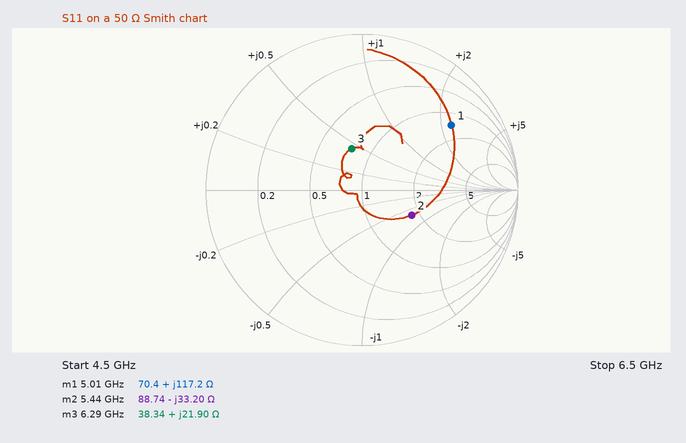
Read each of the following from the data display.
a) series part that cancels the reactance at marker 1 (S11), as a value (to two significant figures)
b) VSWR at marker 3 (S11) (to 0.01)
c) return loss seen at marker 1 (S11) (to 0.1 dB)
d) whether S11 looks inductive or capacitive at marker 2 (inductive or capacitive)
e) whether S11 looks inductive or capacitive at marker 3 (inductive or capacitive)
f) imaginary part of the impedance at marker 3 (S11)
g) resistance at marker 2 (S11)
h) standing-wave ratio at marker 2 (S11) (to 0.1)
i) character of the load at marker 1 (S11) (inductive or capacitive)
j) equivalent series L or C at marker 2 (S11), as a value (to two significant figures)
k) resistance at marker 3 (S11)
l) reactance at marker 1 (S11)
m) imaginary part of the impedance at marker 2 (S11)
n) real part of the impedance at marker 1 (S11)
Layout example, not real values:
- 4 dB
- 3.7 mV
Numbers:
- 270 fF
- 1.75
- 3.0 dB
- capacitive
- inductive
- +21.90 Ω
- 88.74 Ω
- 2.1
- inductive
- 880 fF
- 38.34 Ω
- +117.2 Ω
- -33.20 Ω
- 70.4 Ω
